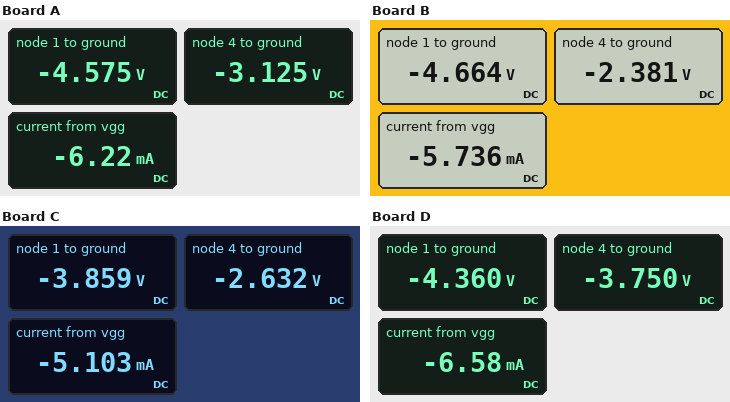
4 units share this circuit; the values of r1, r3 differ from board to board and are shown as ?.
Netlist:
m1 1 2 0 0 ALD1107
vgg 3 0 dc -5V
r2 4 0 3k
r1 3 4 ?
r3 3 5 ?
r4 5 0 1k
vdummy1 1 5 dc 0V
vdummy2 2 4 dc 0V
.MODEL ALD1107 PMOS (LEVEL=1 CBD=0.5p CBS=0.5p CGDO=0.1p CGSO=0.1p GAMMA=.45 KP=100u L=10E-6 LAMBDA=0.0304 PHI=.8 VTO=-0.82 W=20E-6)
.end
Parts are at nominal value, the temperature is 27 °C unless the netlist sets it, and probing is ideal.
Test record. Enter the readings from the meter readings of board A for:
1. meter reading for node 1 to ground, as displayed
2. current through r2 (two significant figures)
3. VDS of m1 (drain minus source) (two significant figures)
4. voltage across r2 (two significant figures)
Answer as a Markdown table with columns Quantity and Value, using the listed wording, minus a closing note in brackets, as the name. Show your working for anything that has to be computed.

| Quantity | Value |
|---|---|
| meter reading for node 1 to ground, as displayed | -4.575 V |
| current through r2 | (0 V - (-3.125 V)) / 3 kΩ = 1.0 mA |
| VDS of m1 (drain minus source) | -4.575 V = -4.6 V |
| voltage across r2 | 0 V - (-3.125 V) = 3.1 V |
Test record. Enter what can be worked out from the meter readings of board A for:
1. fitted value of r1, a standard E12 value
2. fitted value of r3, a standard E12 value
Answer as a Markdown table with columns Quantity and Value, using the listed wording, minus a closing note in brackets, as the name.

| Quantity | Value |
|---|---|
| fitted value of r1, a standard E12 value | 1.8 kΩ |
| fitted value of r3, a standard E12 value | 82 Ω |
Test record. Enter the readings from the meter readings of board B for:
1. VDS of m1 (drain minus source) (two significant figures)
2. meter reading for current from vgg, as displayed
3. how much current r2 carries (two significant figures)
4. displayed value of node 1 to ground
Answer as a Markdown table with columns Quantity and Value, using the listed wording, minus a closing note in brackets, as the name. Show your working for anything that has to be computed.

| Quantity | Value |
|---|---|
| VDS of m1 (drain minus source) | -4.664 V = -4.7 V |
| meter reading for current from vgg, as displayed | -5.736 mA |
| how much current r2 carries | (0 V - (-2.381 V)) / 3 kΩ = 790 µA |
| displayed value of node 1 to ground | -4.664 V |
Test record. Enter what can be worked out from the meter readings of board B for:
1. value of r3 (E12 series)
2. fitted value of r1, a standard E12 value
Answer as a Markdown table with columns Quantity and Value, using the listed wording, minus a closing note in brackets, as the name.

| Quantity | Value |
|---|---|
| value of r3 | 68 Ω |
| fitted value of r1, a standard E12 value | 3.3 kΩ |
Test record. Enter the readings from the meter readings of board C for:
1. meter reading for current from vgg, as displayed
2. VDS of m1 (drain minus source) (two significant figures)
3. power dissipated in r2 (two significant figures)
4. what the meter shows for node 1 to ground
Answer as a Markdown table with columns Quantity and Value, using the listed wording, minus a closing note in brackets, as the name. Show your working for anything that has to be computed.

| Quantity | Value |
|---|---|
| meter reading for current from vgg, as displayed | -5.103 mA |
| VDS of m1 (drain minus source) | -3.859 V = -3.9 V |
| power dissipated in r2 | (0 V - (-2.632 V))^2 / 3 kΩ = 2.3 mW |
| what the meter shows for node 1 to ground | -3.859 V |
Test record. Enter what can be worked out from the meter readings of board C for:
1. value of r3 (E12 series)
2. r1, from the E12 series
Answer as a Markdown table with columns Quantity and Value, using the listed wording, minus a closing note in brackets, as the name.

| Quantity | Value |
|---|---|
| value of r3 | 270 Ω |
| r1, from the E12 series | 2.7 kΩ |
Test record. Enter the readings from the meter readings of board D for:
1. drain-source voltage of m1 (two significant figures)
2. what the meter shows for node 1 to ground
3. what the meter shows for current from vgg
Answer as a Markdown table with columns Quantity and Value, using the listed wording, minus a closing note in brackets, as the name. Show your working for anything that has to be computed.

| Quantity | Value |
|---|---|
| drain-source voltage of m1 | -4.36 V = -4.4 V |
| what the meter shows for node 1 to ground | -4.360 V |
| what the meter shows for current from vgg | -6.58 mA |
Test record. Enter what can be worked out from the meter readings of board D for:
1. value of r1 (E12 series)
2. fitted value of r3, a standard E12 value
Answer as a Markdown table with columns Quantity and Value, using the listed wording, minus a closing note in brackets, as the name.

| Quantity | Value |
|---|---|
| value of r1 | 1 kΩ |
| fitted value of r3, a standard E12 value | 120 Ω |
